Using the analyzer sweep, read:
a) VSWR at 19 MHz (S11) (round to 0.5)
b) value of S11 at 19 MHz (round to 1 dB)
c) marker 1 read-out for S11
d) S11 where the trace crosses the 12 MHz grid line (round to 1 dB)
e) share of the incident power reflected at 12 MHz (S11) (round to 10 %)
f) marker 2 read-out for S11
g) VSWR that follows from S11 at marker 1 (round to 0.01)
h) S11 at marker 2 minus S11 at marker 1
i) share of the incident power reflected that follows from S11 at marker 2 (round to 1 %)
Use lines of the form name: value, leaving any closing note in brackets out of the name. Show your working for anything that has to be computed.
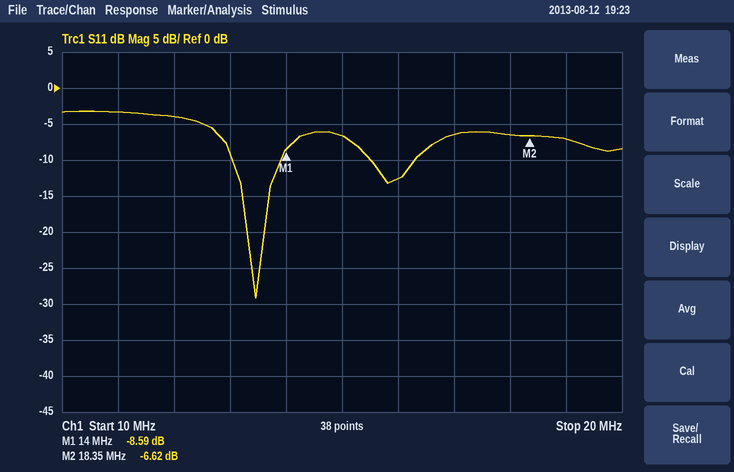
VSWR at 19 MHz (S11): |Γ| = 10^(-7/20) = 0.4467; VSWR = (1 + 0.4467)/(1 − 0.4467) ≈ 2.61, so 2.5 to the nearest 0.5
value of S11 at 19 MHz: -7 dB
marker 1 read-out for S11: -8.59 dB
S11 where the trace crosses the 12 MHz grid line: -4 dB
share of the incident power reflected at 12 MHz (S11): 10^(-4/10) ≈ 40 %
marker 2 read-out for S11: -6.62 dB
VSWR that follows from S11 at marker 1: (1 + 0.3720)/(1 − 0.3720) ≈ 2.18
S11 at marker 2 minus S11 at marker 1: -6.62 − (-8.59) = 1.97 dB
share of the incident power reflected that follows from S11 at marker 2: 10^(-6.62/10) ≈ 22 %
